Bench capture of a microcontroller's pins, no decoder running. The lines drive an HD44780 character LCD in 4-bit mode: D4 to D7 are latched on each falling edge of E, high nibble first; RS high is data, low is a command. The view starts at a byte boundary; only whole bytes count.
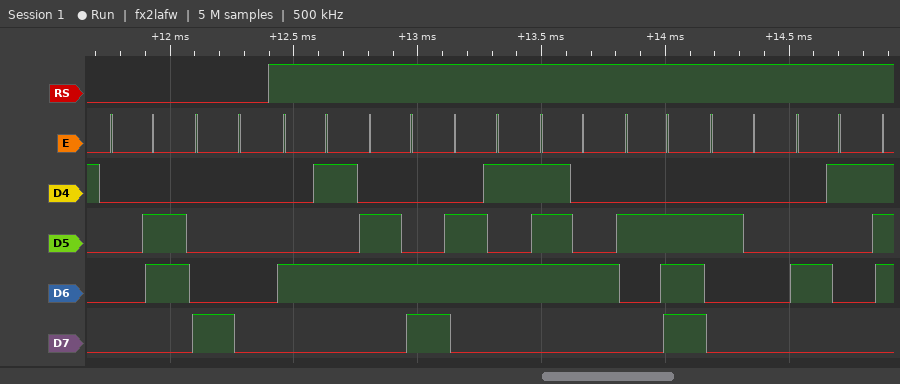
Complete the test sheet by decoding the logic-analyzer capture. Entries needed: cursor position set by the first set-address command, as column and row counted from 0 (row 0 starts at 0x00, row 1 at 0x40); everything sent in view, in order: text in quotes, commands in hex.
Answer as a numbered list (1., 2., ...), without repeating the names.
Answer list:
1. column 0, row 0
2. 0x06 0x80 "Elet. A"
